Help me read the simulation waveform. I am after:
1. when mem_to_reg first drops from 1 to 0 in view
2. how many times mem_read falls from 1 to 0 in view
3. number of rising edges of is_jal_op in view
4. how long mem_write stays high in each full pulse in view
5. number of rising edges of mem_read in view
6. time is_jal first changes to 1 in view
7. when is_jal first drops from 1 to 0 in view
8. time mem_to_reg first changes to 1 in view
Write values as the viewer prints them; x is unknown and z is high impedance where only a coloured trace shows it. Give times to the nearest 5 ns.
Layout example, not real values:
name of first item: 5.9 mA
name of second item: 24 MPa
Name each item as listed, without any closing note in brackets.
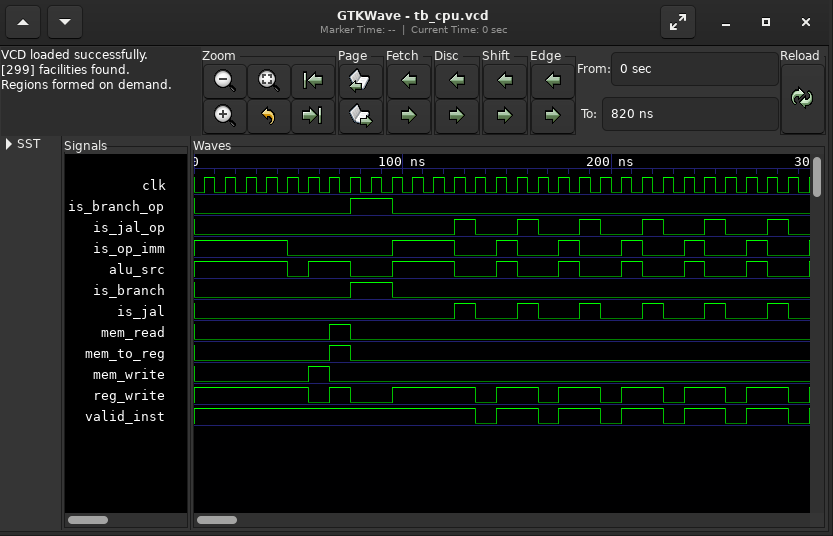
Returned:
when mem_to_reg first drops from 1 to 0 in view: 75 ns
how many times mem_read falls from 1 to 0 in view: 1
number of rising edges of is_jal_op in view: 6
how long mem_write stays high in each full pulse in view: 10 ns
number of rising edges of mem_read in view: 1
time is_jal first changes to 1 in view: 125 ns
when is_jal first drops from 1 to 0 in view: 135 ns
time mem_to_reg first changes to 1 in view: 65 ns
